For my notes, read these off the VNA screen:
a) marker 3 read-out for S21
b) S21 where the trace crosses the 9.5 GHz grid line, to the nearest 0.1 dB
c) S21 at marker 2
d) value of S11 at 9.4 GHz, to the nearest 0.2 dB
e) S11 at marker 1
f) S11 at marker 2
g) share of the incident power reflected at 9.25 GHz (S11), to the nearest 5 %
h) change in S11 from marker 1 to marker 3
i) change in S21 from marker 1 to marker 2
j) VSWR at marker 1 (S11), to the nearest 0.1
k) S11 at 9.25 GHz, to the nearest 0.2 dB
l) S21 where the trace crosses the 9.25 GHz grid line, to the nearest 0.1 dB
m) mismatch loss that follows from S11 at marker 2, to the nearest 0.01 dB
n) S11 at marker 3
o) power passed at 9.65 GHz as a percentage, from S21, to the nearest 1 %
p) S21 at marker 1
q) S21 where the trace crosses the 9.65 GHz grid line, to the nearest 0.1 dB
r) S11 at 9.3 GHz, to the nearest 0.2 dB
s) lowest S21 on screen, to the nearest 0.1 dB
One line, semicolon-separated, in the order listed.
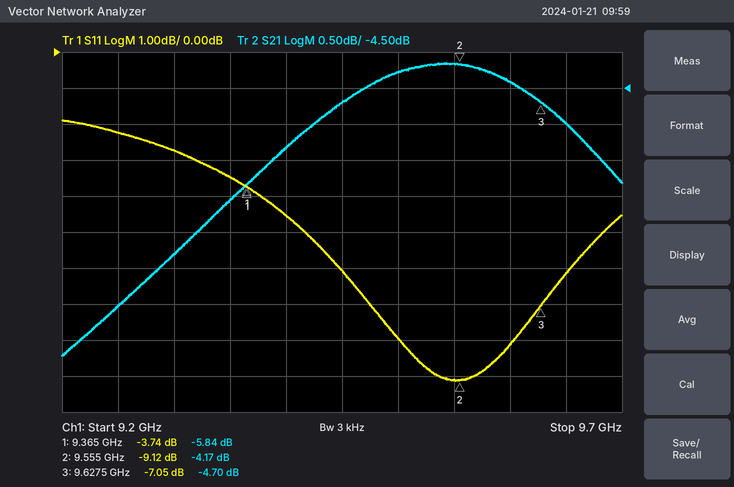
-4.70 dB; -4.3 dB; -4.17 dB; -4.6 dB; -3.74 dB; -9.12 dB; 60 %; -3.31 dB; 1.67 dB; 4.7; -2.2 dB; -7.5 dB; 0.57 dB; -7.05 dB; 32 %; -5.84 dB; -5.0 dB; -2.8 dB; -8.2 dB
